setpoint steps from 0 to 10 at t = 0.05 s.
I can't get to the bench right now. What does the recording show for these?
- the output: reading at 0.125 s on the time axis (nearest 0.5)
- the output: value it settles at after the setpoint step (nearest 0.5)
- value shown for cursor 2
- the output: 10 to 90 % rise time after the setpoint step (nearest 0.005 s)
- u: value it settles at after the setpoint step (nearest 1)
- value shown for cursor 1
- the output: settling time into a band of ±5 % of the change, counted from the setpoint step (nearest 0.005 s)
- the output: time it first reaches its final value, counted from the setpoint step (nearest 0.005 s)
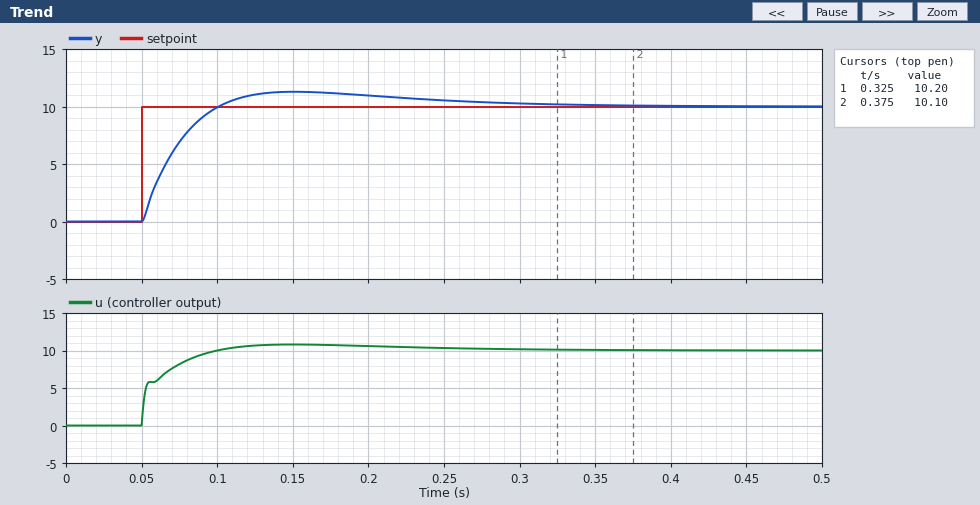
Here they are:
11.0
10.0
10.10
0.035 s
10
10.20
0.205 s
0.050 s
